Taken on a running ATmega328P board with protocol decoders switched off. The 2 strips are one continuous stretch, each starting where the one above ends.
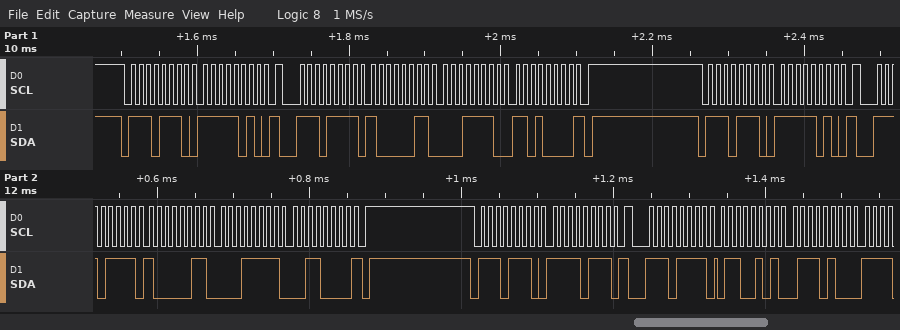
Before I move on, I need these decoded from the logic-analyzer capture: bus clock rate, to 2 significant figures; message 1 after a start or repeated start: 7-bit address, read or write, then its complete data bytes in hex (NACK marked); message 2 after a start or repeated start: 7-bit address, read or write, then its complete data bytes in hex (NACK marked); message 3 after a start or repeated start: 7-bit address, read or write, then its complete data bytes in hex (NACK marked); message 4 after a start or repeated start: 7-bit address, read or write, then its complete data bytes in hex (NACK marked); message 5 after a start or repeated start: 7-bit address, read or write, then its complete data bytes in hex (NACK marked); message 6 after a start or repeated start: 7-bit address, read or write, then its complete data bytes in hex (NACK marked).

100 kHz
0x77 write: FA
0x77 read: 83 1E D0 NACK
0x77 write: FA
0x77 read: 83 1F 30 NACK
0x77 write: F7
0x77 read: 65 74
